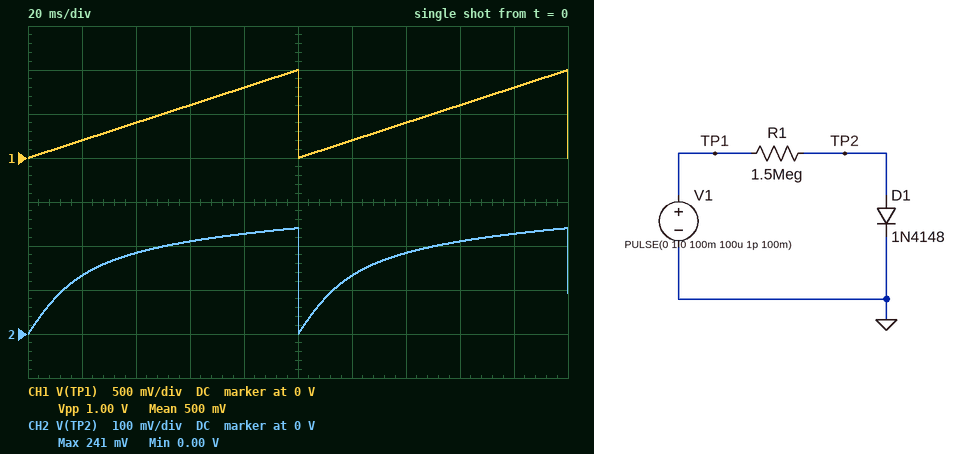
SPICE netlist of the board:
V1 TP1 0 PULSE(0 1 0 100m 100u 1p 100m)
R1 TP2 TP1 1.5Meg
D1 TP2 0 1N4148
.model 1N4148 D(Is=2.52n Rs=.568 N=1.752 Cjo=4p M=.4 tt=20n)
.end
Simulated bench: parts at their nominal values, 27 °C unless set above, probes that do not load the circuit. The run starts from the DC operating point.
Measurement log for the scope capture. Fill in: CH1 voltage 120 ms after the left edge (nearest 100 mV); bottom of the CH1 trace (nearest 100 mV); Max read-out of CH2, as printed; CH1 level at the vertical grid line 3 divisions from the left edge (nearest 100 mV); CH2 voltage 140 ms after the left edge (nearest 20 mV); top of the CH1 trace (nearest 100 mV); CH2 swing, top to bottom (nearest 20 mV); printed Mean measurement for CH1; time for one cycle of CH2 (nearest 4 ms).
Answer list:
200 mV
0 V
241 mV
600 mV
180 mV
1.0 V
240 mV
500 mV
100 ms
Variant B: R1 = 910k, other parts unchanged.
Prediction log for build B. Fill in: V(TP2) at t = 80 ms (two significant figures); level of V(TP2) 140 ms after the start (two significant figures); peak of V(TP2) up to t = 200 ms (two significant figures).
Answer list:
250 mV
200 mV
260 mV
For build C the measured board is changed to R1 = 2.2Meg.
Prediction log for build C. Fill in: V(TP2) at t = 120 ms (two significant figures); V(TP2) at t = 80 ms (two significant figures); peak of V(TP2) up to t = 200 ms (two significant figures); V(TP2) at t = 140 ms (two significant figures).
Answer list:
120 mV
210 mV
220 mV
170 mV
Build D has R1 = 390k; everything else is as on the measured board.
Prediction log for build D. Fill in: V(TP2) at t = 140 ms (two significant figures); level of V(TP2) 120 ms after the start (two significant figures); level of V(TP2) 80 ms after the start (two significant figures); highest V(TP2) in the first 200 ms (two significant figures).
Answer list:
230 mV
160 mV
280 mV
300 mV
